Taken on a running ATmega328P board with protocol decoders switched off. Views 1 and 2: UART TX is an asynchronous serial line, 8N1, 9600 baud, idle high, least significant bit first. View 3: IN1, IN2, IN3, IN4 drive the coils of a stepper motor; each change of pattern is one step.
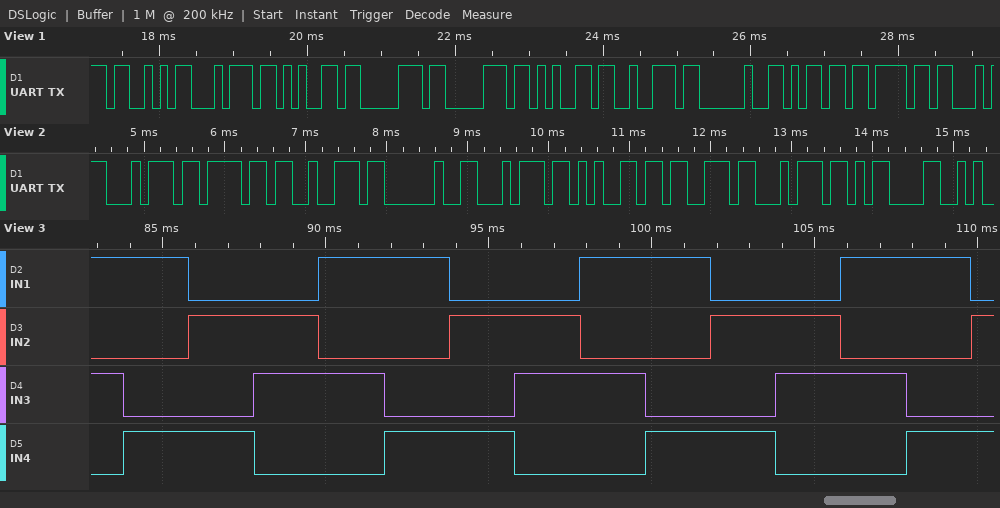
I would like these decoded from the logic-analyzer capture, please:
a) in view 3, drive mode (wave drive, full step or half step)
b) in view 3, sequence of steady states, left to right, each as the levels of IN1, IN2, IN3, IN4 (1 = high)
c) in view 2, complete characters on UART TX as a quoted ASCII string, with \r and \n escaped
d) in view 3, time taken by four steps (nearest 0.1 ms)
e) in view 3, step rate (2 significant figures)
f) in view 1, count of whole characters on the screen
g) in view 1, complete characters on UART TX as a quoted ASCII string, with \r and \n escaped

full step
1010 1001 0101 0110 1010 1001 0101 0110 1010 1001 0101 0110 1010 1001 0101
"tor test\r"
8.0 ms
500 steps/s
10
"Stepper mo"
